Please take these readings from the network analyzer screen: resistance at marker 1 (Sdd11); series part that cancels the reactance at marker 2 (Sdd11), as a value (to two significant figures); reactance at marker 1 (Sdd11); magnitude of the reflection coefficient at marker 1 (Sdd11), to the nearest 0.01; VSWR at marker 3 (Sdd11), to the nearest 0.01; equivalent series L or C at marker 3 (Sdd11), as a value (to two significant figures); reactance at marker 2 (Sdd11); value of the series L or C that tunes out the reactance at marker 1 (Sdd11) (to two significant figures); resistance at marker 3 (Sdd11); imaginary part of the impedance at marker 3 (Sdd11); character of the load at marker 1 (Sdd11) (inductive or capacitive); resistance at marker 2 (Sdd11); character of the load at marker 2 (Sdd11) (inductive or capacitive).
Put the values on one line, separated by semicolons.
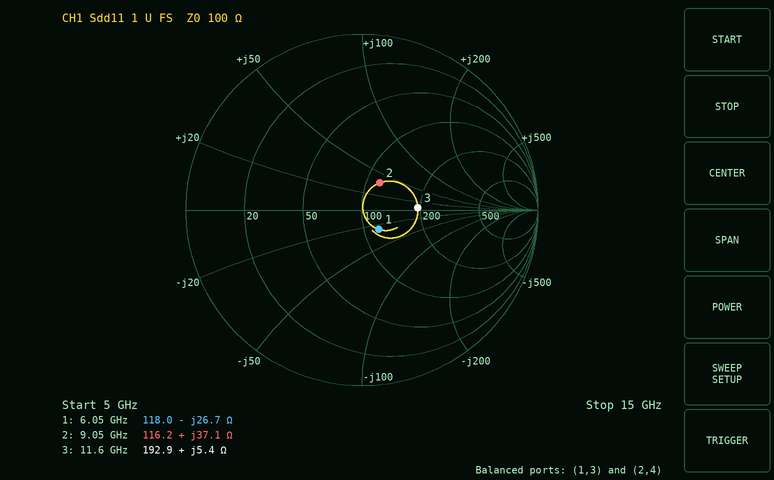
118.0 Ω; 470 fF; -26.7 Ω; 0.15; 1.93; 74 pH; +37.1 Ω; 700 pH; 192.9 Ω; +5.4 Ω; capacitive; 116.2 Ω; inductive
